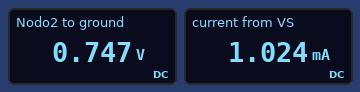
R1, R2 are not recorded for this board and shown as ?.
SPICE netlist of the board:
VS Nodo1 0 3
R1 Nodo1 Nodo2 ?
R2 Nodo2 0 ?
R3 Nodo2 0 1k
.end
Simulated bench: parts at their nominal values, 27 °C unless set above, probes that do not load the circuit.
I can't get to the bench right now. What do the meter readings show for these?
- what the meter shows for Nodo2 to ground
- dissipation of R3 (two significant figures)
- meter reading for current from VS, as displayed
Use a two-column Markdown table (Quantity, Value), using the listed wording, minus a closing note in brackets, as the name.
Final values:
| Quantity | Value |
|---|---|
| what the meter shows for Nodo2 to ground | 0.747 V |
| dissipation of R3 | 560 µW |
| meter reading for current from VS, as displayed | 1.024 mA |
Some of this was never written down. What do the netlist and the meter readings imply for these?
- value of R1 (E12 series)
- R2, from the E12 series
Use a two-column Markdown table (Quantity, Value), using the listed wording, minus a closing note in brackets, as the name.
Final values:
| Quantity | Value |
|---|---|
| value of R1 | 2.2 kΩ |
| R2, from the E12 series | 2.7 kΩ |
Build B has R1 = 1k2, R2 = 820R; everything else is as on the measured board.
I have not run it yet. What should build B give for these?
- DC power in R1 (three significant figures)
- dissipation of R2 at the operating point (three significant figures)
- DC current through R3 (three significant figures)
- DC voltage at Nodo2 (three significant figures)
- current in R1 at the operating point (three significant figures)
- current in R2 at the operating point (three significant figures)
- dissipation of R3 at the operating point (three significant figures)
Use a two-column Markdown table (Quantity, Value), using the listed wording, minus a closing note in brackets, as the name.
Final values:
| Quantity | Value |
|---|---|
| DC power in R1 | 3.96 mW |
| dissipation of R2 at the operating point | 818 µW |
| DC current through R3 | 819 µA |
| DC voltage at Nodo2 | 819 mV |
| current in R1 at the operating point | 1.82 mA |
| current in R2 at the operating point | 999 µA |
| dissipation of R3 at the operating point | 671 µW |
